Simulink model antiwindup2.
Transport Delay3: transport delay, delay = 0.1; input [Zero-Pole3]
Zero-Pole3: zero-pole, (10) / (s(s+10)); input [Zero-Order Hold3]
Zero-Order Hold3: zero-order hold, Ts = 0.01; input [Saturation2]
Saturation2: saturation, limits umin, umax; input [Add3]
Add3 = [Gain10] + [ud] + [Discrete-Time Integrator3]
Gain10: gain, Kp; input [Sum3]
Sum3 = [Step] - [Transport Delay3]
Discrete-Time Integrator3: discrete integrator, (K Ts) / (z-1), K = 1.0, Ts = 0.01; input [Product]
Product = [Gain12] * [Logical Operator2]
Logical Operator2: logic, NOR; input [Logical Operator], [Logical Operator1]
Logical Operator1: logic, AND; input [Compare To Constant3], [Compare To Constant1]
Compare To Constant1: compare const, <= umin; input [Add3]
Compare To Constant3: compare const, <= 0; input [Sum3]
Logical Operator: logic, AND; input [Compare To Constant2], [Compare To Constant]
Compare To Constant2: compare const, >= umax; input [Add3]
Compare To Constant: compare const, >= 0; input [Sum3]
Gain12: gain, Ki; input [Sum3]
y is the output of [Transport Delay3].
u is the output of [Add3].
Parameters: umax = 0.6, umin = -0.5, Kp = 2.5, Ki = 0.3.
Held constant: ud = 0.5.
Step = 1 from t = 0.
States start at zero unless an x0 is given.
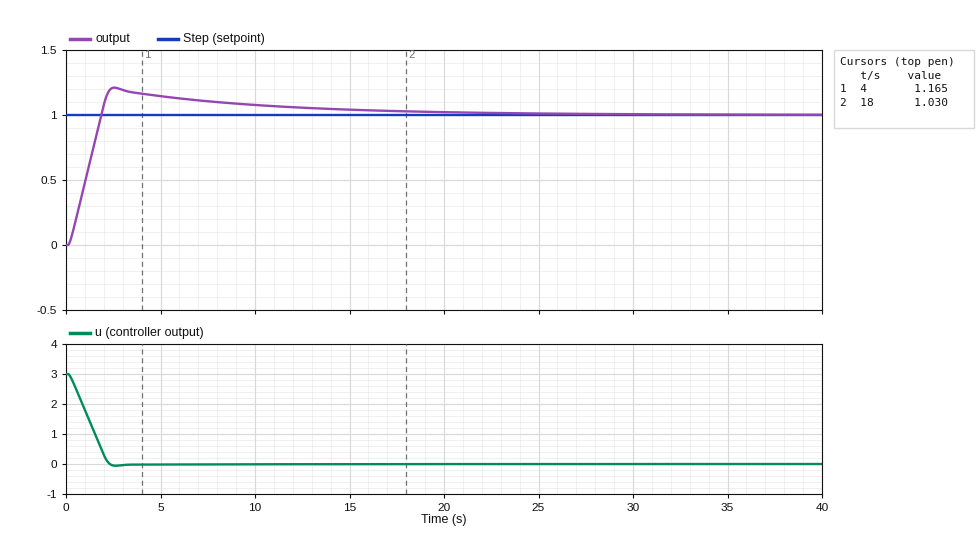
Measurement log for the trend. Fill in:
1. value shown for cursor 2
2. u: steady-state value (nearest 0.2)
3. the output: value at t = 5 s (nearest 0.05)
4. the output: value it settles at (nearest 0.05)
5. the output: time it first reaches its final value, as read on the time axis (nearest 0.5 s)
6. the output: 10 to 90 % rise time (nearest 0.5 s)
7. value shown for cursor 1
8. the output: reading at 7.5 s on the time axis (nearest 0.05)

1.030
0.0
1.15
1.00
2.0 s
1.5 s
1.165
1.10
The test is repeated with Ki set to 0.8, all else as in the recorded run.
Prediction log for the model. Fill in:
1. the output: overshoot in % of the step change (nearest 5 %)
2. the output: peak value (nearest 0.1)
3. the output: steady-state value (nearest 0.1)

20 %
1.2
1.0
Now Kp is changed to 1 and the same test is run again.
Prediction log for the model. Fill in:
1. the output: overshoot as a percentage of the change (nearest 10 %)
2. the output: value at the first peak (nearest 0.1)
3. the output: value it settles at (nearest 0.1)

40 %
1.4
1.0
